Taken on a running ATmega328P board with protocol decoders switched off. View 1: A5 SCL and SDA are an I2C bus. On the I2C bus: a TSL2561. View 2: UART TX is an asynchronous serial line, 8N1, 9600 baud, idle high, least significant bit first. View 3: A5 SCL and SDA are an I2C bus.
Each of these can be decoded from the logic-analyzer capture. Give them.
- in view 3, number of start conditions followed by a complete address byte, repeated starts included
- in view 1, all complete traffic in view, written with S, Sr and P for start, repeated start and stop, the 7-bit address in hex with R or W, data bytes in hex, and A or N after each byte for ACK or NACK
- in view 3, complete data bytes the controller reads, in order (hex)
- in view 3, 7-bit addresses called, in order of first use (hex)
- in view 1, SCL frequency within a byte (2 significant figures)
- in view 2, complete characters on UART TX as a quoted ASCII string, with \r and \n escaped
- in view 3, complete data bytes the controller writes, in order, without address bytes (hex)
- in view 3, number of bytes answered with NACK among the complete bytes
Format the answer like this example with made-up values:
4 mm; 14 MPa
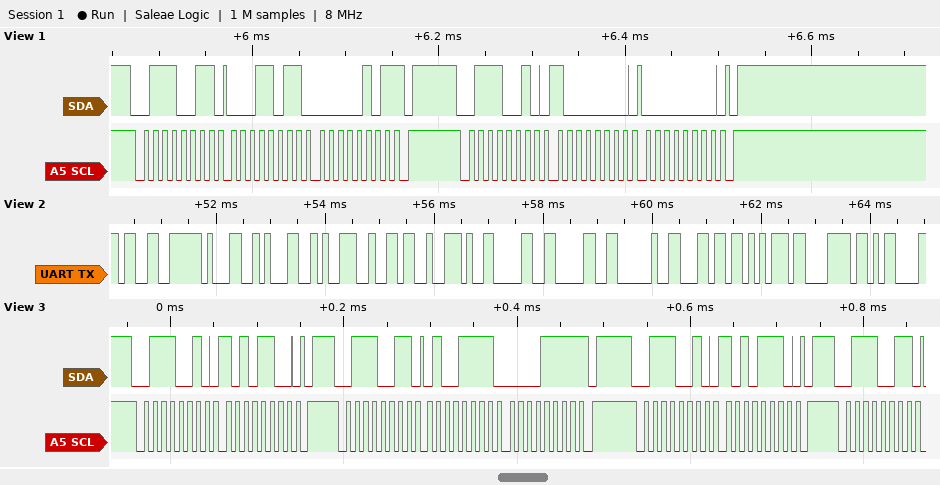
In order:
4; S 39R A 1B A 05 N P S 39W A 80 A 00 A P; 4F 0F; 0x39; 100 kHz; "31196.00 lux\r"; AC AE; 1
